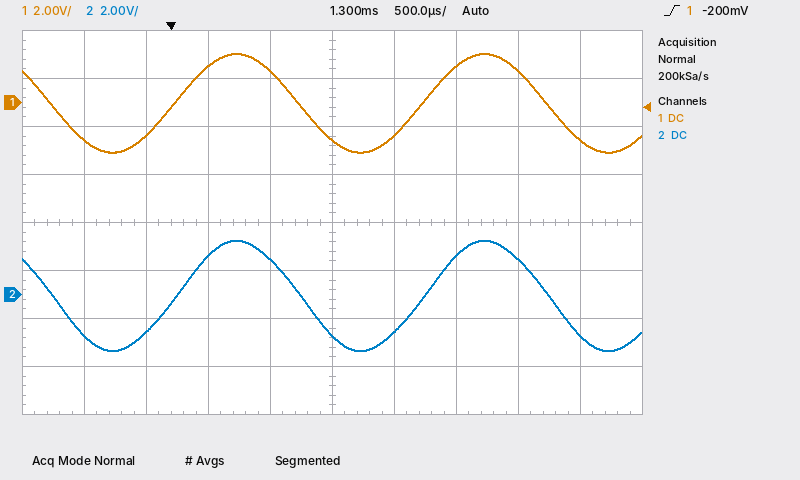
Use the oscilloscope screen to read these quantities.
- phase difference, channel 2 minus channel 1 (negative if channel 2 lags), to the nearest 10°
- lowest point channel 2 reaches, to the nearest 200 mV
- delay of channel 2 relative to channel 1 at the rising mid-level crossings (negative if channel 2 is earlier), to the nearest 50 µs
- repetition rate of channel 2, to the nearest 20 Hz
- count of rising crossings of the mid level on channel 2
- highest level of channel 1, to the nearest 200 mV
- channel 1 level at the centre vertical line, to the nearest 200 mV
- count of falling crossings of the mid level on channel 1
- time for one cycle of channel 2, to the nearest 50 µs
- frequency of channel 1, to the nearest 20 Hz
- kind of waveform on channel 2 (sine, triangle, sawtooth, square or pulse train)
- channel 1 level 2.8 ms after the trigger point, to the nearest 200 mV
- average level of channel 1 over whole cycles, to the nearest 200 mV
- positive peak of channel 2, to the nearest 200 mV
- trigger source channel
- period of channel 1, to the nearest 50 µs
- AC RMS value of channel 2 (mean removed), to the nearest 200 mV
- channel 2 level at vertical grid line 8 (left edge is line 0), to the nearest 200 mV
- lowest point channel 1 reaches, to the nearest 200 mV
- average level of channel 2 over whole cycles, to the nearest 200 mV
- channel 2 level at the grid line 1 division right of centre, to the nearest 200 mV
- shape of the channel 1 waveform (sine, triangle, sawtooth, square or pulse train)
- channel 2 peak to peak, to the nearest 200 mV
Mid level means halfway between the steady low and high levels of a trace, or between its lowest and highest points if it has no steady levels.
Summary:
0°
-2.4 V
0 µs
500 Hz
2
2.0 V
-1.6 V
3
2.00 ms
500 Hz
sine
1.4 V
0.0 V
2.2 V
channel 1
2.00 ms
1.6 V
1.4 V
-2.0 V
0.0 V
-1.6 V
sine
4.6 V
